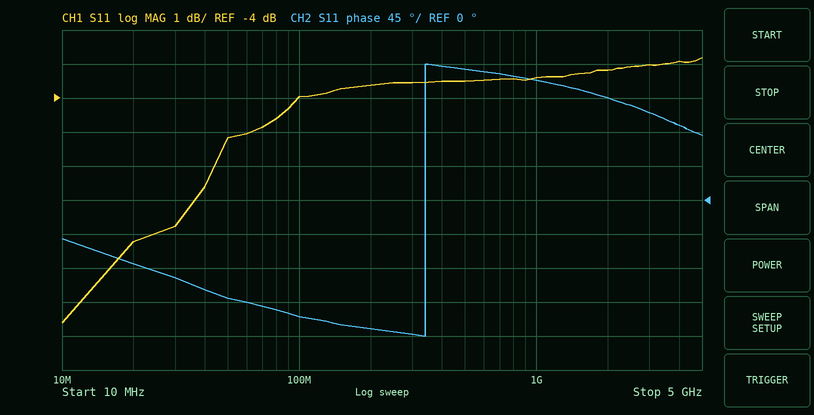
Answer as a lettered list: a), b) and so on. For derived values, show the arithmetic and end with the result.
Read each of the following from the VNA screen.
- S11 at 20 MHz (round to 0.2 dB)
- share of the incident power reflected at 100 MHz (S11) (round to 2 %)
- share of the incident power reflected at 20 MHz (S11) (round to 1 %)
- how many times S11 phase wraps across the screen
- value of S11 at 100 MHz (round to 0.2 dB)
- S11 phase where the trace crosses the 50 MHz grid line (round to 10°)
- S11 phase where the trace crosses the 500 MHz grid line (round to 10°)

a) -8.2 dB
b) 10^(-4/10) ≈ 40 %
c) 10^(-8.2/10) ≈ 15 %
d) 1
e) -4.0 dB
f) -130°
g) 170°
